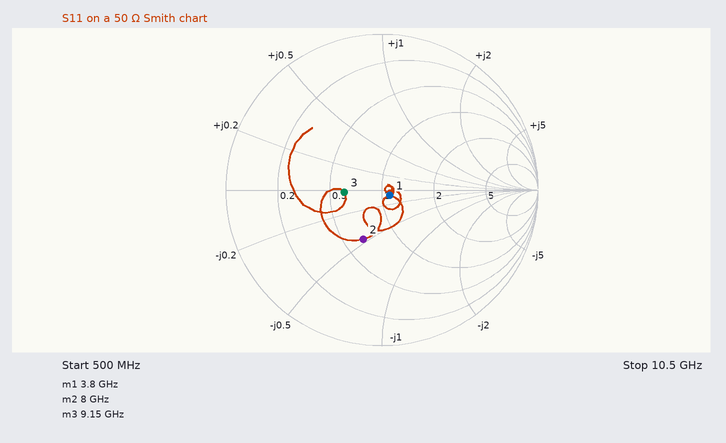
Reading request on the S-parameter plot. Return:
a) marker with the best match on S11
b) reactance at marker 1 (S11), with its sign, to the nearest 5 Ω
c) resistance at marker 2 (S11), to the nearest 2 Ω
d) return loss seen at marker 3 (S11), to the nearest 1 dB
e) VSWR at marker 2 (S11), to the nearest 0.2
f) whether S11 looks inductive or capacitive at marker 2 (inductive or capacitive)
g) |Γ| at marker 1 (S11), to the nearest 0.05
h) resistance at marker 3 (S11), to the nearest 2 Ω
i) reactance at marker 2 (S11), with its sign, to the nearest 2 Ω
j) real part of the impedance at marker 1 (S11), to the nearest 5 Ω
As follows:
marker 1
-5 Ω
32 Ω
12 dB
2.0
capacitive
0.05
30 Ω
-24 Ω
55 Ω
